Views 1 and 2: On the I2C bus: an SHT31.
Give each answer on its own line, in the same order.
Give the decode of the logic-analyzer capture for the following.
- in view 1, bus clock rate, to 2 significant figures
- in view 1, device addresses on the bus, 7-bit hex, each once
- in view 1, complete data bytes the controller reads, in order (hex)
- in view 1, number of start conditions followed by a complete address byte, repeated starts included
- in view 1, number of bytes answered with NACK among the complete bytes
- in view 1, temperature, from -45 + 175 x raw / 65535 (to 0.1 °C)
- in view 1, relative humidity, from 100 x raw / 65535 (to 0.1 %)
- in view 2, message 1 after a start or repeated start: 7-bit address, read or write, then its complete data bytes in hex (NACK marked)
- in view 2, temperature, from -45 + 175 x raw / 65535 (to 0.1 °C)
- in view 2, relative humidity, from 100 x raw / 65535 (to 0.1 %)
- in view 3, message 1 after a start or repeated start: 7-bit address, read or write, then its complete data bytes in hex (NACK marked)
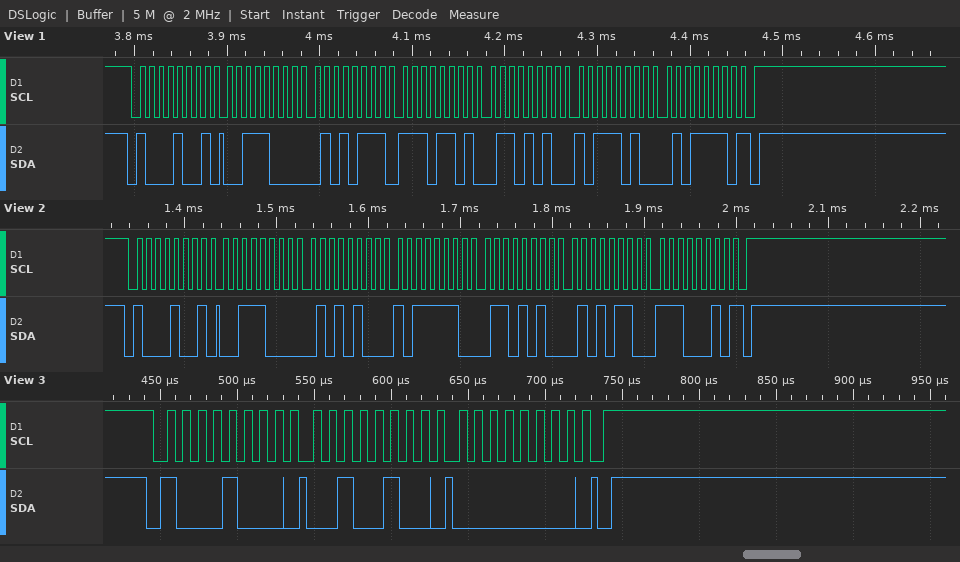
100 kHz
0x44
38 57 ED 6A BA 5E
1
1
-6.5 °C
41.7 %
0x44 read: 38 54 BE 6A 56 E2 NACK
-6.5 °C
41.5 %
0x44 write: 24 00
